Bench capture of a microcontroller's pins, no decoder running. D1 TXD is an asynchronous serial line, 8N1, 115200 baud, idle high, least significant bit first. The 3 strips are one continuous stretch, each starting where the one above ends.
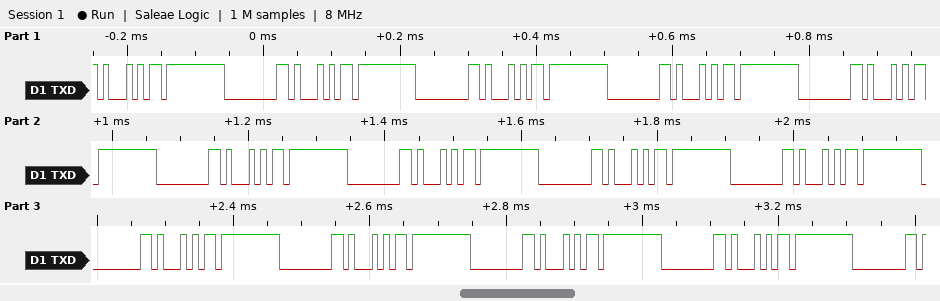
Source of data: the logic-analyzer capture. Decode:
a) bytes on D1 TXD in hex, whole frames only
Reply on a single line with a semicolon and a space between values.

51 FF 00 51 FF 00 51 FF 00 51 FF 00 51 FF 00 51 FF 00 51 FF 00 51 FF 00 51 FF 00 51 FF 00 51 FF 00 51 FF 00 51 FF 00
